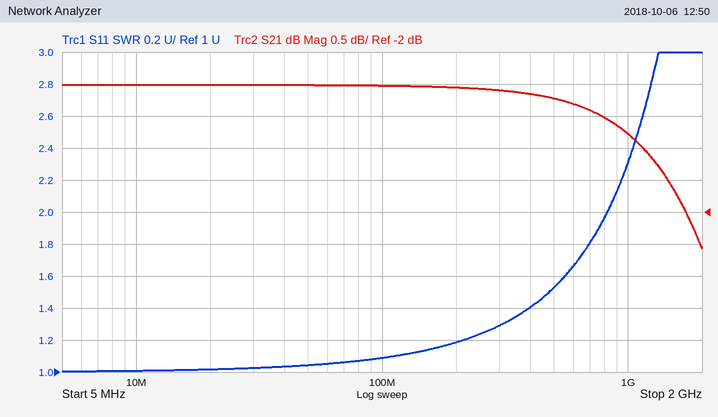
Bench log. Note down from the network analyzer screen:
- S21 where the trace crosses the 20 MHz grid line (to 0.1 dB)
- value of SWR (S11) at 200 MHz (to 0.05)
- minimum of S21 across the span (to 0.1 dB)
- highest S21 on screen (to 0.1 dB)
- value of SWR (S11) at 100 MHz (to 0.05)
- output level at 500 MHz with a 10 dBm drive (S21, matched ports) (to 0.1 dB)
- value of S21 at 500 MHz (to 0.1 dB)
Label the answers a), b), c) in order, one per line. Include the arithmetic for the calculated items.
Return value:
a) 0.0 dB
b) 1.20
c) -2.6 dB
d) 0.0 dB
e) 1.10
f) 10 dBm + (-0.2 dB) = 9.8 dBm
g) -0.2 dB
